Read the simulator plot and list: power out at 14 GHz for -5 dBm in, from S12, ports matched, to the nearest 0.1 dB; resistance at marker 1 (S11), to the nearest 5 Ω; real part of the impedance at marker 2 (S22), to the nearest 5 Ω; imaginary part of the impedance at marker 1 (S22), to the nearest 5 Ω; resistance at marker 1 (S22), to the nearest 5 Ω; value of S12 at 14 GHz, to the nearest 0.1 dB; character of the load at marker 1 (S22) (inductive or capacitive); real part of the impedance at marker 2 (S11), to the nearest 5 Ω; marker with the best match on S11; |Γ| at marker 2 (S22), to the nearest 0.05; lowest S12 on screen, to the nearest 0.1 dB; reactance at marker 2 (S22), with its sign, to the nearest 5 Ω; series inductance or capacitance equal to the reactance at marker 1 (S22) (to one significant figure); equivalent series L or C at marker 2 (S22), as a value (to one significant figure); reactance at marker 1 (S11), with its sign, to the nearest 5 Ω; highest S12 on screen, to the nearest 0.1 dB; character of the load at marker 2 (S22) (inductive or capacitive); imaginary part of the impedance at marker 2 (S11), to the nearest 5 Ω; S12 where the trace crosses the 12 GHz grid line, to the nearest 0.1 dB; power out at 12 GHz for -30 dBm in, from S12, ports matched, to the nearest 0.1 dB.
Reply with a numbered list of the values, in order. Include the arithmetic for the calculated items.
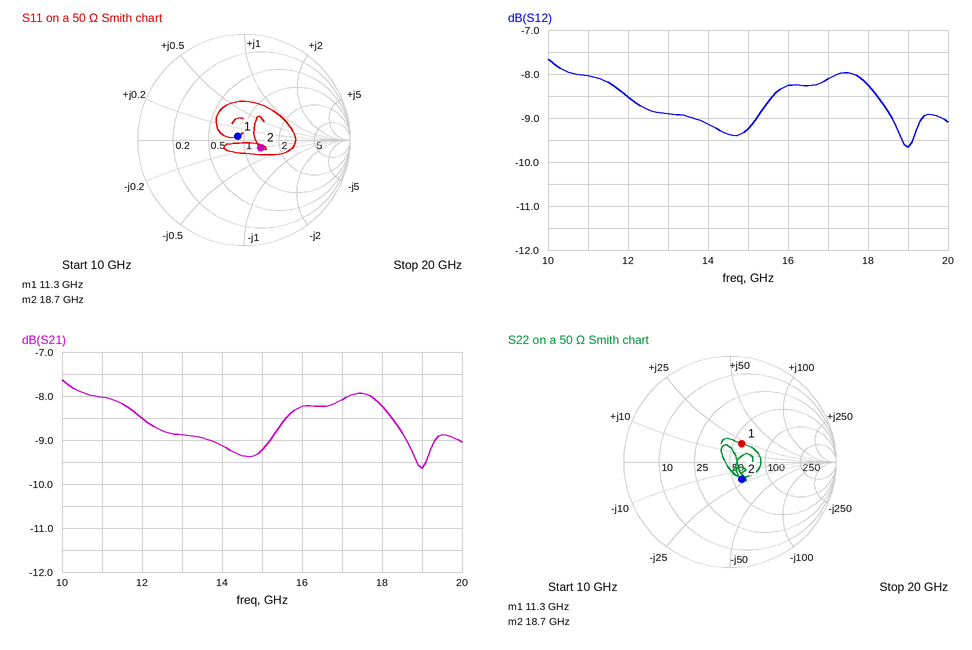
1. -5 dBm + (-9.1 dB) = -14.1 dBm
2. 45 Ω
3. 60 Ω
4. +20 Ω
5. 60 Ω
6. -9.1 dB
7. inductive
8. 70 Ω
9. marker 1
10. 0.20
11. -9.7 dB
12. -20 Ω
13. L = 20 Ω/(2π × 11.3 GHz) ≈ 282 pH, so 300 pH to one significant figure
14. C = 1/(2π × 18.7 GHz × 20 Ω) ≈ 426 fF, so 400 fF to one significant figure
15. +5 Ω
16. -7.7 dB
17. capacitive
18. -10 Ω
19. -8.5 dB
20. -30 dBm + (-8.5 dB) = -38.5 dBm
